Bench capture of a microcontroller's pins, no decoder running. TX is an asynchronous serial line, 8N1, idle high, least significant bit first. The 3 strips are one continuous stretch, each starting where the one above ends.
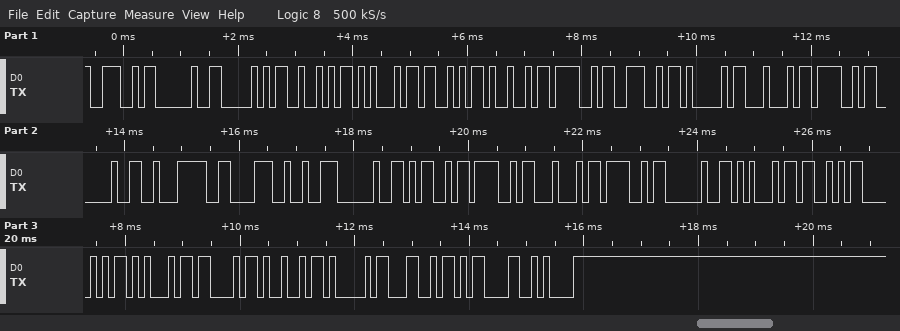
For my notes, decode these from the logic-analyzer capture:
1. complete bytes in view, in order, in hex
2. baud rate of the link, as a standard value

4E 20 50 52 45 53 49 4F 4E 41 44 4F 20 E2 86 92 20 4D 4F 44 4F 20 45 53 50 45 43 49 41 4C 0D 0A
9600 baud
